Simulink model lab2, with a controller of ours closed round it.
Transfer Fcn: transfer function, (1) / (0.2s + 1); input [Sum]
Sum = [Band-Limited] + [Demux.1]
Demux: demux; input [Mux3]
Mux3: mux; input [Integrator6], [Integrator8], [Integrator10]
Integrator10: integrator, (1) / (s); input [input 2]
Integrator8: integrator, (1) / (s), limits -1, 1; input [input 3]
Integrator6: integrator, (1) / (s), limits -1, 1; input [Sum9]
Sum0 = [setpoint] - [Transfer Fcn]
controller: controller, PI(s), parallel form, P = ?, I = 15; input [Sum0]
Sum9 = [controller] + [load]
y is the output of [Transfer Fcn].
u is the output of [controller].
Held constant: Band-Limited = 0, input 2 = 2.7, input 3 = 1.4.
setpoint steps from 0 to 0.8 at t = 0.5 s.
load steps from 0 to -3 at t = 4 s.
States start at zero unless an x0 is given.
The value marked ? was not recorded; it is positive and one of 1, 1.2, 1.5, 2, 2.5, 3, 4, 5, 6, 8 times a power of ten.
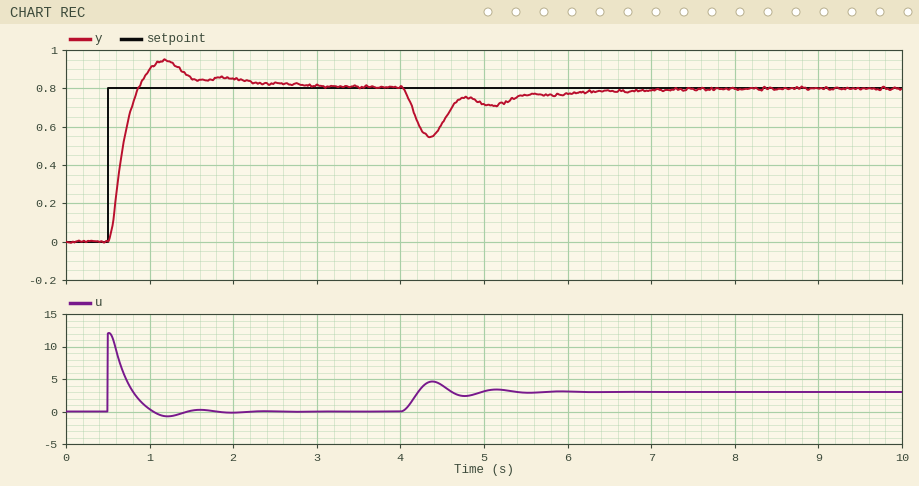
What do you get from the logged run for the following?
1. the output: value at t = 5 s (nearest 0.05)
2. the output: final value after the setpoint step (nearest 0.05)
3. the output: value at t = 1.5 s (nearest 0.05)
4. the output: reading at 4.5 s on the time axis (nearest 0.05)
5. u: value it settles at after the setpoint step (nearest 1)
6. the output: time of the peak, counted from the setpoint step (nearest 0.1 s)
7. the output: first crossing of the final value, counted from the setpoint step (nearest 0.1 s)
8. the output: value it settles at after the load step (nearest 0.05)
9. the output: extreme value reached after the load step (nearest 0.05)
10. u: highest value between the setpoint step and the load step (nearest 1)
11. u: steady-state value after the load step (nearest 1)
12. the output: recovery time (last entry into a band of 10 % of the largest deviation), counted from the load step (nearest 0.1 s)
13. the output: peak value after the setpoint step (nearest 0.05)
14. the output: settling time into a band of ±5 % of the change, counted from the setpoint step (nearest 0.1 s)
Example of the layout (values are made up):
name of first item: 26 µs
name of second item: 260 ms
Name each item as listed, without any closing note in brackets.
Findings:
the output: value at t = 5 s: 0.70
the output: final value after the setpoint step: 0.80
the output: value at t = 1.5 s: 0.85
the output: reading at 4.5 s on the time axis: 0.60
u: value it settles at after the setpoint step: 0
the output: time of the peak, counted from the setpoint step: 0.7 s
the output: first crossing of the final value, counted from the setpoint step: 0.4 s
the output: value it settles at after the load step: 0.80
the output: extreme value reached after the load step: 0.55
u: highest value between the setpoint step and the load step: 12
u: steady-state value after the load step: 3
the output: recovery time (last entry into a band of 10 % of the largest deviation), counted from the load step: 2.1 s
the output: peak value after the setpoint step: 0.95
the output: settling time into a band of ±5 % of the change, counted from the setpoint step: 1.6 s
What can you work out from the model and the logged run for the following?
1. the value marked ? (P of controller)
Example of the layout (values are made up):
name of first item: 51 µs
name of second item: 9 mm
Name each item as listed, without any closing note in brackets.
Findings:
the value marked ?: 15
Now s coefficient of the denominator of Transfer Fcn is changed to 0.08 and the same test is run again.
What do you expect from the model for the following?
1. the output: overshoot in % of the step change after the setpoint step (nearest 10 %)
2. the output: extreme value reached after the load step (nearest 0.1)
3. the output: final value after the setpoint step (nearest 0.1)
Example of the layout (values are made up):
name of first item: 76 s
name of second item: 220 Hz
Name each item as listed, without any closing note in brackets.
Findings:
the output: overshoot in % of the step change after the setpoint step: 20 %
the output: extreme value reached after the load step: 0.6
the output: final value after the setpoint step: 0.8
